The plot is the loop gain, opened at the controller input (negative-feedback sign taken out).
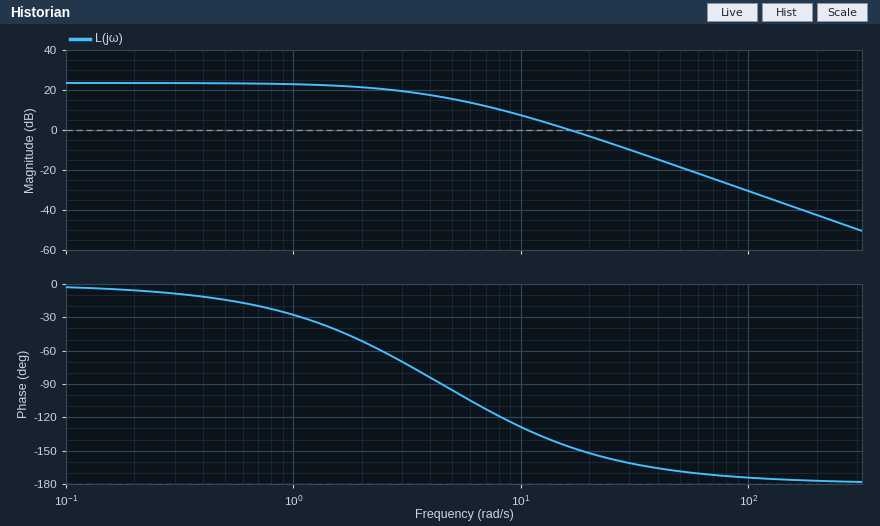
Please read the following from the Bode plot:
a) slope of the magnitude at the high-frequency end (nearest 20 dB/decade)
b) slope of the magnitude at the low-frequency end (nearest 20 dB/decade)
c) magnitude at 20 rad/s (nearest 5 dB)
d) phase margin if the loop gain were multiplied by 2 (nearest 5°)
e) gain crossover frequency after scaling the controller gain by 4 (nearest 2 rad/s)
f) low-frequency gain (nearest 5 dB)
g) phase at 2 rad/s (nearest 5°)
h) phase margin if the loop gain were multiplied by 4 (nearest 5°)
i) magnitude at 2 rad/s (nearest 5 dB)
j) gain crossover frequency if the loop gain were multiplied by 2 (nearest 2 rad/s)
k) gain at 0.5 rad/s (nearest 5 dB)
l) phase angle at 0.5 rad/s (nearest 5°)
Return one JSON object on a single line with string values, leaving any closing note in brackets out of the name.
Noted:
{"slope of the magnitude at the high-frequency end": "-40 dB/decade", "slope of the magnitude at the low-frequency end": "0 dB/decade", "magnitude at 20 rad/s": "-5 dB", "phase margin if the loop gain were multiplied by 2": "25°", "gain crossover frequency after scaling the controller gain by 4": "34 rad/s", "low-frequency gain": "25 dB", "phase at 2 rad/s": "-50°", "phase margin if the loop gain were multiplied by 4": "15°", "magnitude at 2 rad/s": "20 dB", "gain crossover frequency if the loop gain were multiplied by 2": "24 rad/s", "gain at 0.5 rad/s": "25 dB", "phase angle at 0.5 rad/s": "-15°"}
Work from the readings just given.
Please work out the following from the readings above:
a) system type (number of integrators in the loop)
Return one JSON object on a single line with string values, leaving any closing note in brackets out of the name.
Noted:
{"system type": "0"}
